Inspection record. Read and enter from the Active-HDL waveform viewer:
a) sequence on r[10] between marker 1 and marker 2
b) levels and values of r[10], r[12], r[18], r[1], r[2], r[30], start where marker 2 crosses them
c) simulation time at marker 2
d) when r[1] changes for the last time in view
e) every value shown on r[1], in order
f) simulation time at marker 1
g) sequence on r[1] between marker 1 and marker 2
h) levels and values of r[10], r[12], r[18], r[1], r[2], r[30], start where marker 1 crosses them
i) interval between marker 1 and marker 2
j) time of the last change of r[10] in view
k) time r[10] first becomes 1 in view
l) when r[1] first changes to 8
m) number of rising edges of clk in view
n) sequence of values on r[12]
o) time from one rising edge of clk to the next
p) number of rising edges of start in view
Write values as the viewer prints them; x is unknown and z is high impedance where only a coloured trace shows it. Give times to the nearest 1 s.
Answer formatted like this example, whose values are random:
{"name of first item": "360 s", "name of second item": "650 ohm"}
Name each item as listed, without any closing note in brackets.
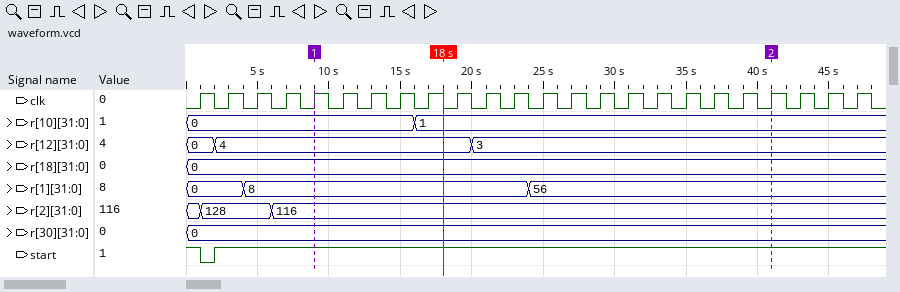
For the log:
{"sequence on r[10] between marker 1 and marker 2": "0, 1", "levels and values of r[10], r[12], r[18], r[1], r[2], r[30], start where marker 2 crosses them": "r[10]=1, r[12]=3, r[18]=0, r[1]=56, r[2]=116, r[30]=0, start=1", "simulation time at marker 2": "41 s", "when r[1] changes for the last time in view": "24 s", "every value shown on r[1], in order": "0, 8, 56", "simulation time at marker 1": "9 s", "sequence on r[1] between marker 1 and marker 2": "8, 56", "levels and values of r[10], r[12], r[18], r[1], r[2], r[30], start where marker 1 crosses them": "r[10]=0, r[12]=4, r[18]=0, r[1]=8, r[2]=116, r[30]=0, start=1", "interval between marker 1 and marker 2": "32 s", "time of the last change of r[10] in view": "16 s", "time r[10] first becomes 1 in view": "16 s", "when r[1] first changes to 8": "4 s", "number of rising edges of clk in view": "24", "sequence of values on r[12]": "0, 4, 3", "time from one rising edge of clk to the next": "2 s", "number of rising edges of start in view": "1"}
